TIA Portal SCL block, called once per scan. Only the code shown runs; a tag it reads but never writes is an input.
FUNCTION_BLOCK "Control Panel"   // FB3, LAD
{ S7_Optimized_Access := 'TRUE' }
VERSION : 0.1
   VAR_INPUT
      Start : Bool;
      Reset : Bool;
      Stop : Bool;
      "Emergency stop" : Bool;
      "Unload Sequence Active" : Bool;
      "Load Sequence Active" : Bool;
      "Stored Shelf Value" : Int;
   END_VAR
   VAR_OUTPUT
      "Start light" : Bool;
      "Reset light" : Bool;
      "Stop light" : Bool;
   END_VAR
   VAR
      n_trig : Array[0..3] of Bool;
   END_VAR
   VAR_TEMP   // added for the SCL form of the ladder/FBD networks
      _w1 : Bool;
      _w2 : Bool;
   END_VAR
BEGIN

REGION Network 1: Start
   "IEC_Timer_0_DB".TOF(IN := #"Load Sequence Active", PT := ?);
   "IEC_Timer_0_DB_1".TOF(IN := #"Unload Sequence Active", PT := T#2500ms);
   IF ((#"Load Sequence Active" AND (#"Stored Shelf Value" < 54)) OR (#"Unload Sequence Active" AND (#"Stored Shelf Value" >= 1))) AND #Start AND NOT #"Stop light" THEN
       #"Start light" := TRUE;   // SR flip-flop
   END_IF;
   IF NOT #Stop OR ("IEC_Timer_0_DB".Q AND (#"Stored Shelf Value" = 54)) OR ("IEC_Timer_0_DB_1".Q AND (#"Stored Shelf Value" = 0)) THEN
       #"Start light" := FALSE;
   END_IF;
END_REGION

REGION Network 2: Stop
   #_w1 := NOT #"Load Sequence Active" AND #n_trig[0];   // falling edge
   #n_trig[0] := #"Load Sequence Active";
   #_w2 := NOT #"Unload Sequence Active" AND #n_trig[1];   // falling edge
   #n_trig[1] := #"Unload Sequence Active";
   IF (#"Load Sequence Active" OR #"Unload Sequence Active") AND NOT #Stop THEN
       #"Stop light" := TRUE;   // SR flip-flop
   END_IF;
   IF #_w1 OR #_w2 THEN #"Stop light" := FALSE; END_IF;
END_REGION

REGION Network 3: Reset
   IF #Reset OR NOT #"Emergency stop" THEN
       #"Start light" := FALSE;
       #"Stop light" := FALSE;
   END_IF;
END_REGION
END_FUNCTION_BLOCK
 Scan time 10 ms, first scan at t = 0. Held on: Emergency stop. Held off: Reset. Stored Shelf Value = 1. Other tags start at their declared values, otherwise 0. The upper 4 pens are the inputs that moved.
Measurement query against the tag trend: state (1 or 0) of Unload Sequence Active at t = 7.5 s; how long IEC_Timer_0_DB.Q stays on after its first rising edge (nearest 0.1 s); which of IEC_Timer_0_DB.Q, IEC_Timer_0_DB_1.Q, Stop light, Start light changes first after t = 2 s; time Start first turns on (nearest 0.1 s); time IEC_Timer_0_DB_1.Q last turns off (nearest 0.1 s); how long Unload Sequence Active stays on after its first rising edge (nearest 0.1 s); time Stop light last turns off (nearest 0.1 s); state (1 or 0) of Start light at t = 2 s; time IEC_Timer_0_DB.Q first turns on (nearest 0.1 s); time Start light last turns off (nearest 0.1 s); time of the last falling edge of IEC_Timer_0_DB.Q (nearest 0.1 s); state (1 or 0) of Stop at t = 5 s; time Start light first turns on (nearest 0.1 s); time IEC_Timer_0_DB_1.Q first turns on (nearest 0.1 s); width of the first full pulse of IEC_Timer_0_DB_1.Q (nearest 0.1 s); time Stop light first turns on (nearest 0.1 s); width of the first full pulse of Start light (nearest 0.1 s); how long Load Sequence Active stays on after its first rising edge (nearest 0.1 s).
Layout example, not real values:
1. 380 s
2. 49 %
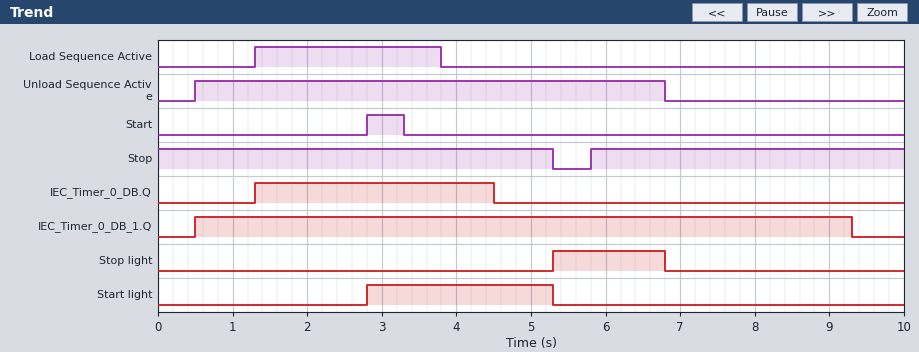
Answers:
1. 0
2. 3.2 s
3. Start light
4. 2.8 s
5. 9.3 s
6. 6.3 s
7. 6.8 s
8. 0
9. 1.3 s
10. 5.3 s
11. 4.5 s
12. 1
13. 2.8 s
14. 0.5 s
15. 8.8 s
16. 5.3 s
17. 2.5 s
18. 2.5 s
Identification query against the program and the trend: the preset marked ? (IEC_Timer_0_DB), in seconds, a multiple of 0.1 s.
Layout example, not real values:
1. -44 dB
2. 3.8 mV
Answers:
1. 0.7 s
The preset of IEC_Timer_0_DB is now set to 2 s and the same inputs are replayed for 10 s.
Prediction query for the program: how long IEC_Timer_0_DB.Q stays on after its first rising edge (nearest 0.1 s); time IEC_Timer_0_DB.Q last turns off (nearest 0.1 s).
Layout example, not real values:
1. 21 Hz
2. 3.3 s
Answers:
1. 4.5 s
2. 5.8 s
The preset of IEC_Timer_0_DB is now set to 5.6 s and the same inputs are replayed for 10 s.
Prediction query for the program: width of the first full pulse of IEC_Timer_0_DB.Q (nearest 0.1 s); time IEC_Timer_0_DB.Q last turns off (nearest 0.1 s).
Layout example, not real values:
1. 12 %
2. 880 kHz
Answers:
1. 8.1 s
2. 9.4 s
